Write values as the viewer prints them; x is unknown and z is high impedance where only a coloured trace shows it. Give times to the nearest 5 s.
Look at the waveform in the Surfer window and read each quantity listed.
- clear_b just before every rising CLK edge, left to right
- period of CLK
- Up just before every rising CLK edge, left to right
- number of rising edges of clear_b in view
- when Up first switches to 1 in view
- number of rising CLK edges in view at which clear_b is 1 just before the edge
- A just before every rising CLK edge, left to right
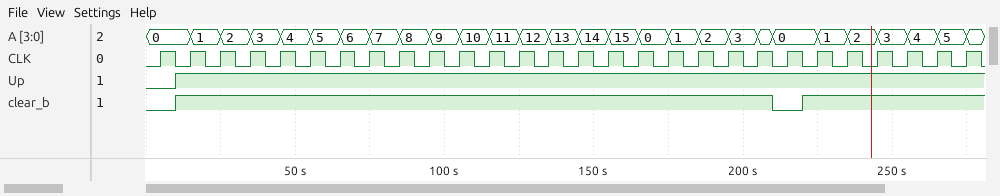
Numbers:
0 1 1 1 1 1 1 1 1 1 1 1 1 1 1 1 1 1 1 1 1 0 1 1 1 1 1 1
10 s
0 1 1 1 1 1 1 1 1 1 1 1 1 1 1 1 1 1 1 1 1 1 1 1 1 1 1 1
2
10 s
26
0, 0, 1, 2, 3, 4, 5, 6, 7, 8, 9, 10, 11, 12, 13, 14, 15, 0, 1, 2, 3, 0, 0, 1, 2, 3, 4, 5
